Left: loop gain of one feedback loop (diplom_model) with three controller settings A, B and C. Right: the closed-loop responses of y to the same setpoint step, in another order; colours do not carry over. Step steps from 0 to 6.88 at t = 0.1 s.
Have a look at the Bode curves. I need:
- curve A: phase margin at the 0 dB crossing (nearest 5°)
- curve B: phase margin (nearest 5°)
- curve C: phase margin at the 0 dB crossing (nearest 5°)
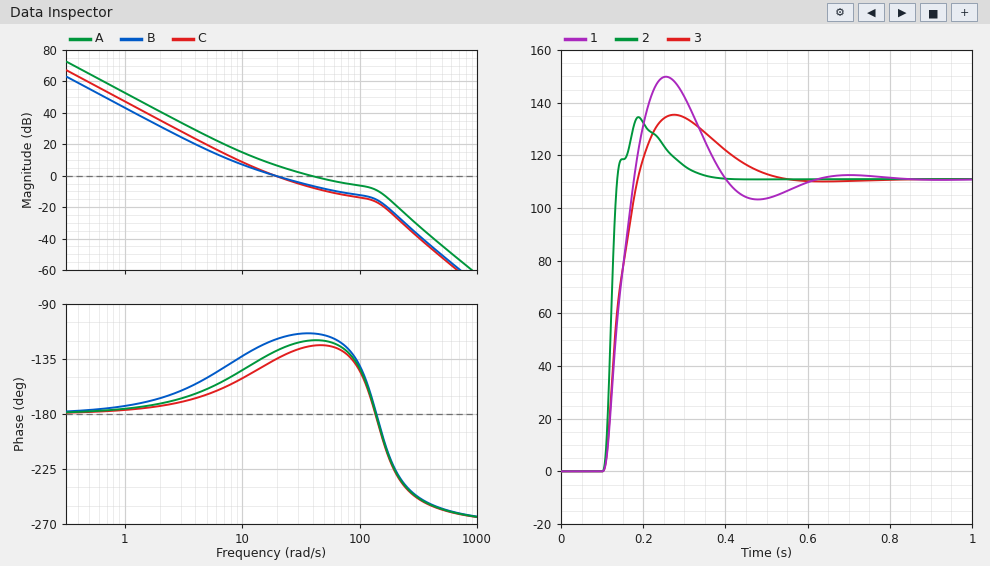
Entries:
60°
60°
45°
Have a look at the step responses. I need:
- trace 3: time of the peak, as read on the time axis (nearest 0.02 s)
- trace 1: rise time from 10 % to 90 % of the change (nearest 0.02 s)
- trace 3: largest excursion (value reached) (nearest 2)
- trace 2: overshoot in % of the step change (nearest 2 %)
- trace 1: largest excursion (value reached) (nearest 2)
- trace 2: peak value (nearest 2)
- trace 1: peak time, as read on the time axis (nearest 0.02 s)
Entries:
0.28 s
0.06 s
136
22 %
150
134
0.26 s
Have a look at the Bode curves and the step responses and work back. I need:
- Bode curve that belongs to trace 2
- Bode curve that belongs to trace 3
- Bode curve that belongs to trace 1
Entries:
A
B
C
